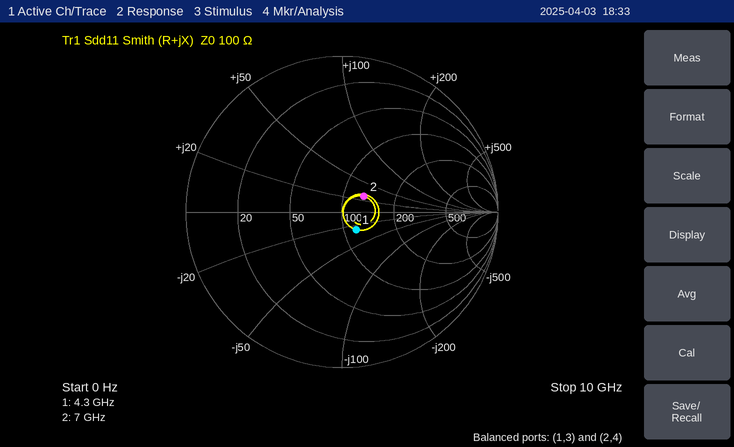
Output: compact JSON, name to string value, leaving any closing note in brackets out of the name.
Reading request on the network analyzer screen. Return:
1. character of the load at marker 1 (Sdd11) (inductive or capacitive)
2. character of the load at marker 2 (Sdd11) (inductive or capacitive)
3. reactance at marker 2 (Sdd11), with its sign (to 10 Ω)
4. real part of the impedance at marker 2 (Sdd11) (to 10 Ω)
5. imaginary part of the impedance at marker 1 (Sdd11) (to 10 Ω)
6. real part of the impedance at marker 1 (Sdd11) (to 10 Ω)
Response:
{"character of the load at marker 1 (Sdd11)": "capacitive", "character of the load at marker 2 (Sdd11)": "inductive", "reactance at marker 2 (Sdd11), with its sign": "+30 Ω", "real part of the impedance at marker 2 (Sdd11)": "130 Ω", "imaginary part of the impedance at marker 1 (Sdd11)": "-30 Ω", "real part of the impedance at marker 1 (Sdd11)": "120 Ω"}
